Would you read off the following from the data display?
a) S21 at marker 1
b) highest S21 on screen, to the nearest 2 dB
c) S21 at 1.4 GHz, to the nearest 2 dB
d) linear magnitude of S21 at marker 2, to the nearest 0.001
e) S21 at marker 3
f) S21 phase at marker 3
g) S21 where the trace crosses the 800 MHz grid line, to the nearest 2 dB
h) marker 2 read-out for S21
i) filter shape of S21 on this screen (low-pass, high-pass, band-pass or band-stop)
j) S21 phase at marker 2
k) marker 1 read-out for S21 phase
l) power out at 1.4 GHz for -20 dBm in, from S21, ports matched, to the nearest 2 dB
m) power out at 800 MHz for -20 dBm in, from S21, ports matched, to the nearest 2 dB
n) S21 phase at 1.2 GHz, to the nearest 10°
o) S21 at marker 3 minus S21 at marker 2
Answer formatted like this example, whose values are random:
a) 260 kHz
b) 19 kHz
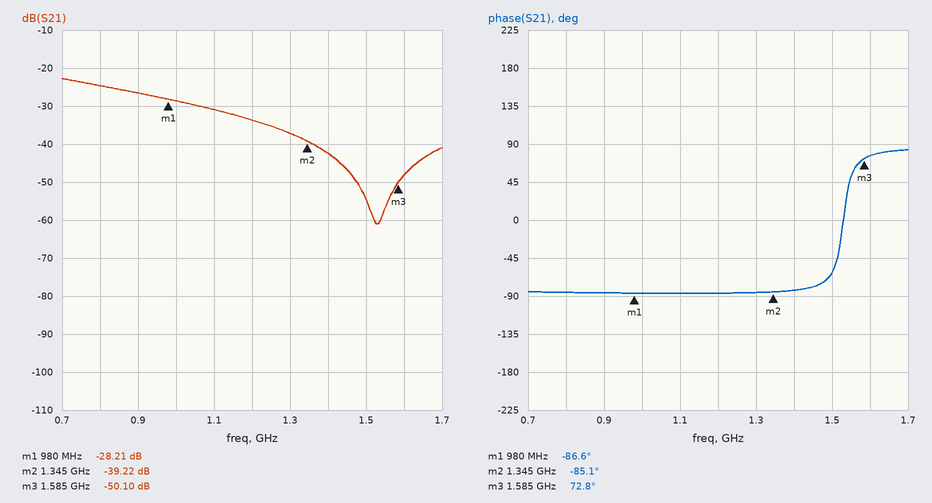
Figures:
a) -28.21 dB
b) -22 dB
c) -42 dB
d) 0.011
e) -50.10 dB
f) 72.8°
g) -24 dB
h) -39.22 dB
i) low-pass
j) -85.1°
k) -86.6°
l) -62 dBm
m) -44 dBm
n) -90°
o) -10.88 dB
